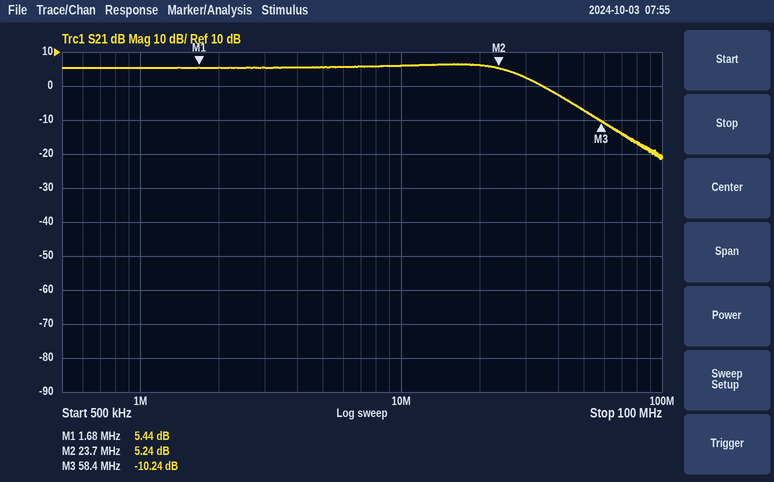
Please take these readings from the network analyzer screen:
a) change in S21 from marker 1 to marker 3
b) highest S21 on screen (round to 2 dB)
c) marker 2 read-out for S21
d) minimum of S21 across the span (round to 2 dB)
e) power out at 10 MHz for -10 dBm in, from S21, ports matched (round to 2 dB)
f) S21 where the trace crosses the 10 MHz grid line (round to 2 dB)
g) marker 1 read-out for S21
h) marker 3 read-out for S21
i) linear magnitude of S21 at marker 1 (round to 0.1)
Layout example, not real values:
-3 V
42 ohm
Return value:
-15.68 dB
6 dB
5.24 dB
-22 dB
-4 dBm
6 dB
5.44 dB
-10.24 dB
1.9
